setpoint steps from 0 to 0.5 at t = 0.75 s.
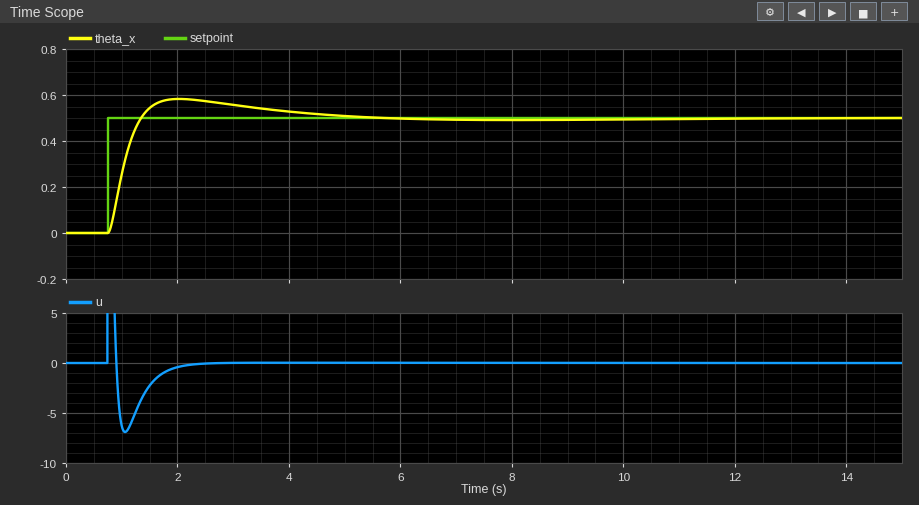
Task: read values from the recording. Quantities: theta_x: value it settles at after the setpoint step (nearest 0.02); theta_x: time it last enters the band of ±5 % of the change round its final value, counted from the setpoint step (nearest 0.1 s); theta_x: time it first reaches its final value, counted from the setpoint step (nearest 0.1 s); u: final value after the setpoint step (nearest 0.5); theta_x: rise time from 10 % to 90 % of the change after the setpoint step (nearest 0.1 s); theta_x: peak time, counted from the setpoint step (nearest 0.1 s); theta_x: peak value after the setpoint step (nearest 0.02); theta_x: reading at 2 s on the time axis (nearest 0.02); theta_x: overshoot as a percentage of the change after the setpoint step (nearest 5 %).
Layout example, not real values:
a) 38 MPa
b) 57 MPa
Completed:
a) 0.50
b) 3.4 s
c) 0.6 s
d) 0.0
e) 0.4 s
f) 1.3 s
g) 0.58
h) 0.58
i) 15 %
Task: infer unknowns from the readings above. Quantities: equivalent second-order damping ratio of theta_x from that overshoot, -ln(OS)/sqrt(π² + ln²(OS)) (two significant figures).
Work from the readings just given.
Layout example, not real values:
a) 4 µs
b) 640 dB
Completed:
a) 0.52
